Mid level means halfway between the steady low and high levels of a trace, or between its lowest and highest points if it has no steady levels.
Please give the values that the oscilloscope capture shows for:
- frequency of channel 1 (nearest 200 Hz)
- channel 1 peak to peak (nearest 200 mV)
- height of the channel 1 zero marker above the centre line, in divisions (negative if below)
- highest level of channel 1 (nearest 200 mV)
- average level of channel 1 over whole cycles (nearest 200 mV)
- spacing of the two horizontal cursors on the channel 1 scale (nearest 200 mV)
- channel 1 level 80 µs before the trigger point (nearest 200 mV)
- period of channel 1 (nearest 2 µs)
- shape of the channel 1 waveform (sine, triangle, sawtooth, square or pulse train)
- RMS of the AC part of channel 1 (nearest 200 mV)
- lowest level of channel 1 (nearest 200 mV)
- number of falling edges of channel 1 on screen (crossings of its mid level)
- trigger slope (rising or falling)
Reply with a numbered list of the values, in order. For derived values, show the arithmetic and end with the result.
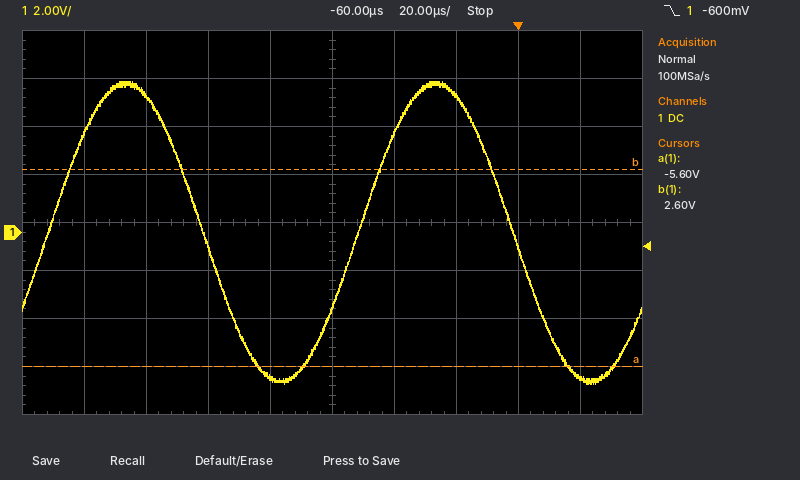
1. 1 / 100 µs ≈ 10.0 kHz
2. 6.2 V − (-6.4 V) = 12.6 V
3. -0.2 div
4. 6.2 V
5. (6.2 V + (-6.4 V)) / 2 ≈ 0.0 V
6. 8.2 V
7. -6.0 V
8. 100 µs
9. sine
10. 12.6 V / (2√2) ≈ 4.4 V
11. -6.4 V
12. 2
13. falling
